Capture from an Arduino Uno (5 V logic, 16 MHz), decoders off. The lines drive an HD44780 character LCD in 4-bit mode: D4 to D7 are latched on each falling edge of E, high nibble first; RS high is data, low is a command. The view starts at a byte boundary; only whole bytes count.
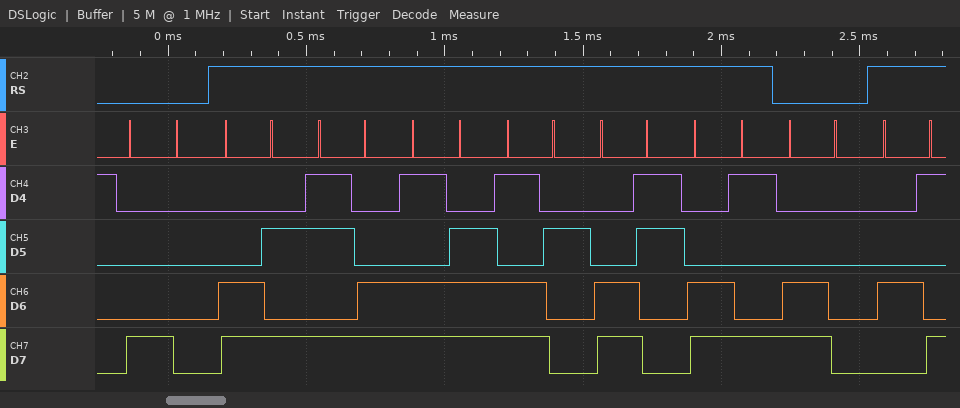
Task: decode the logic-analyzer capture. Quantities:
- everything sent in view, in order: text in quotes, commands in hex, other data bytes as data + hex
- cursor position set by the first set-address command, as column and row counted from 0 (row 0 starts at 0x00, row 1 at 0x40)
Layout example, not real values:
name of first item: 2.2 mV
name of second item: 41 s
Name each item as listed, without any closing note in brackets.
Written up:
everything sent in view, in order: text in quotes, commands in hex, other data bytes as data + hex: 0x80 data CA BC DE D2 C3 C9 0xC0 "I"
cursor position set by the first set-address command, as column and row counted from 0: column 0, row 0
